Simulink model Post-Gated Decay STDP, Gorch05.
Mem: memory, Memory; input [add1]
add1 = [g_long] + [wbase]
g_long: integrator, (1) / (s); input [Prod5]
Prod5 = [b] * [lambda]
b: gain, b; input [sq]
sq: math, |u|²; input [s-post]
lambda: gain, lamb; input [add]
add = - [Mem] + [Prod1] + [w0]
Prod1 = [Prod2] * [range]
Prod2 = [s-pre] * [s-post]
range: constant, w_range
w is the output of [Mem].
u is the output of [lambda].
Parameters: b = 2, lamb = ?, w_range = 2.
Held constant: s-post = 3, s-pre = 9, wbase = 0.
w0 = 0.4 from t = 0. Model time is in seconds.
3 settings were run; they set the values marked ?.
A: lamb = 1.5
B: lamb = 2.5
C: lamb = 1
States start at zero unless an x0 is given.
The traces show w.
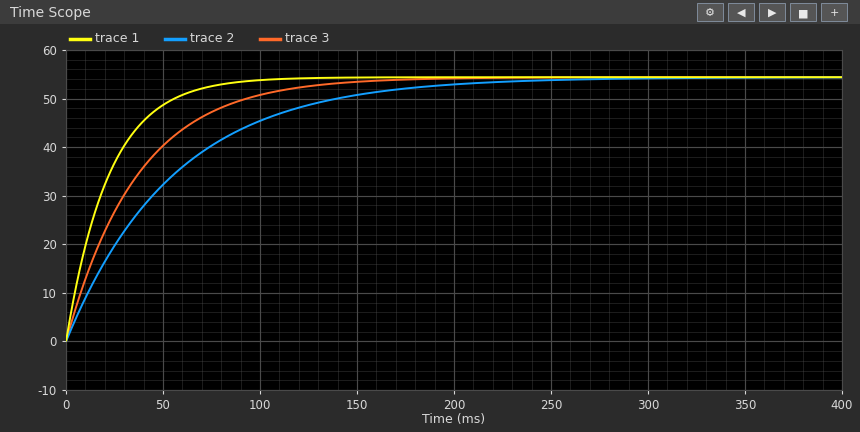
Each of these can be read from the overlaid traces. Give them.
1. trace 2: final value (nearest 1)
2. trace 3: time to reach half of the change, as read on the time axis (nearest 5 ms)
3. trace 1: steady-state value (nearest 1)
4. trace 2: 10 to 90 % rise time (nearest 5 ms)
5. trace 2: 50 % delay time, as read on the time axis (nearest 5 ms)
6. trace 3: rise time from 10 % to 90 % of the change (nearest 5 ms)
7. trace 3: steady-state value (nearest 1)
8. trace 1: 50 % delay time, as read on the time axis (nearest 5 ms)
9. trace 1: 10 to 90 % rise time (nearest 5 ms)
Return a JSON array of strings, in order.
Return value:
["54", "25 ms", "54", "120 ms", "40 ms", "80 ms", "54", "15 ms", "50 ms"]
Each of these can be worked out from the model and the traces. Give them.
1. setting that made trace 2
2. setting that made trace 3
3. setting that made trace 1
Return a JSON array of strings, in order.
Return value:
["C", "A", "B"]
